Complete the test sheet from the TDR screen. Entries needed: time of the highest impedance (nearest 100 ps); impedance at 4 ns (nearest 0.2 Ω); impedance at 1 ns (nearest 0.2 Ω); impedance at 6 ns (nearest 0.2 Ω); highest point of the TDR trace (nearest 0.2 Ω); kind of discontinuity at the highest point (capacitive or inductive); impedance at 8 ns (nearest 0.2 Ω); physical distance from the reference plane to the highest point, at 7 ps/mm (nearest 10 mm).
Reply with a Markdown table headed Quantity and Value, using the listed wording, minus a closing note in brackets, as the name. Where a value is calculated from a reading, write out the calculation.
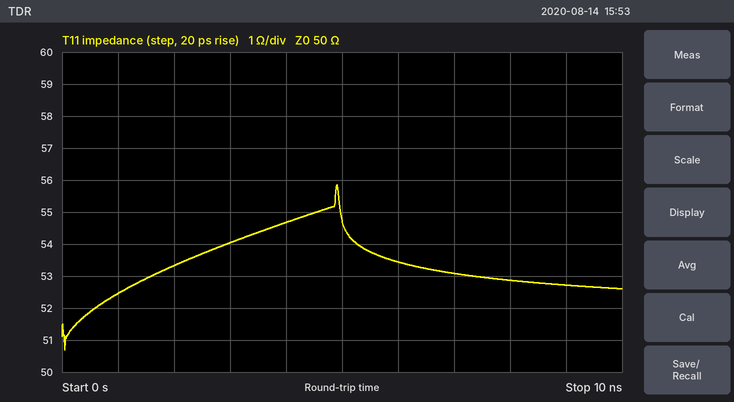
| Quantity | Value |
|---|---|
| time of the highest impedance | 4.9 ns |
| impedance at 4 ns | 54.6 Ω |
| impedance at 1 ns | 52.4 Ω |
| impedance at 6 ns | 53.4 Ω |
| highest point of the TDR trace | 55.8 Ω |
| kind of discontinuity at the highest point | inductive |
| impedance at 8 ns | 52.8 Ω |
| physical distance from the reference plane to the highest point, at 7 ps/mm | 4.9 ns / 2 / 7 ps/mm ≈ 350 mm |
